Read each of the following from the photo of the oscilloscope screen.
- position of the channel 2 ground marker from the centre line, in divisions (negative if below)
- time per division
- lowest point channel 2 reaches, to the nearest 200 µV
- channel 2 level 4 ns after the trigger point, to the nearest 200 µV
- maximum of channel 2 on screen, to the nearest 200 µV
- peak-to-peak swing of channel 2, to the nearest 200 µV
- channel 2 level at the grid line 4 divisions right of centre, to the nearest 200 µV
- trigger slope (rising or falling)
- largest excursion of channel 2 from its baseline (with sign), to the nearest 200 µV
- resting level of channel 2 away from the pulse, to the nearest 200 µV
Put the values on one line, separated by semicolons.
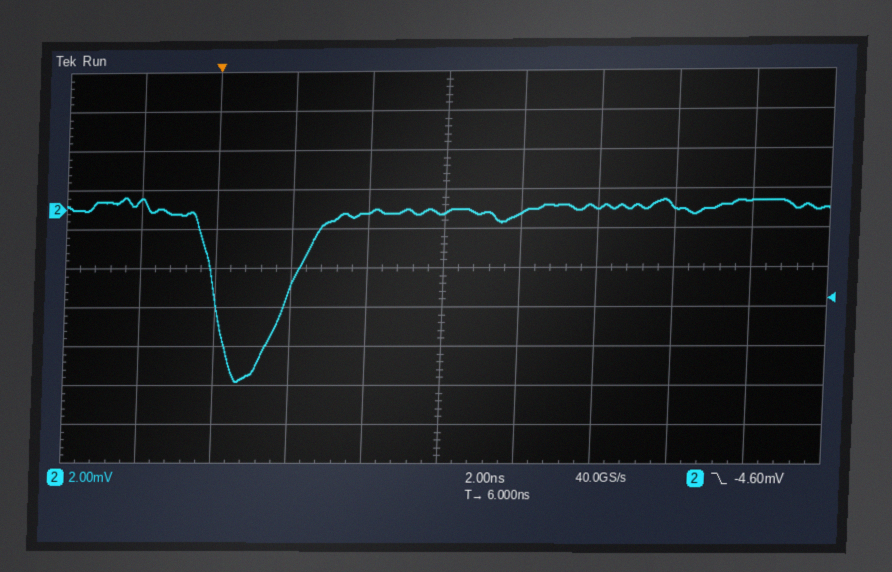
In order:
+1.5 div; 2 ns; -8.8 mV; -200 µV; 600 µV; 9.4 mV; 400 µV; falling; -8.8 mV; 0.0 mV
